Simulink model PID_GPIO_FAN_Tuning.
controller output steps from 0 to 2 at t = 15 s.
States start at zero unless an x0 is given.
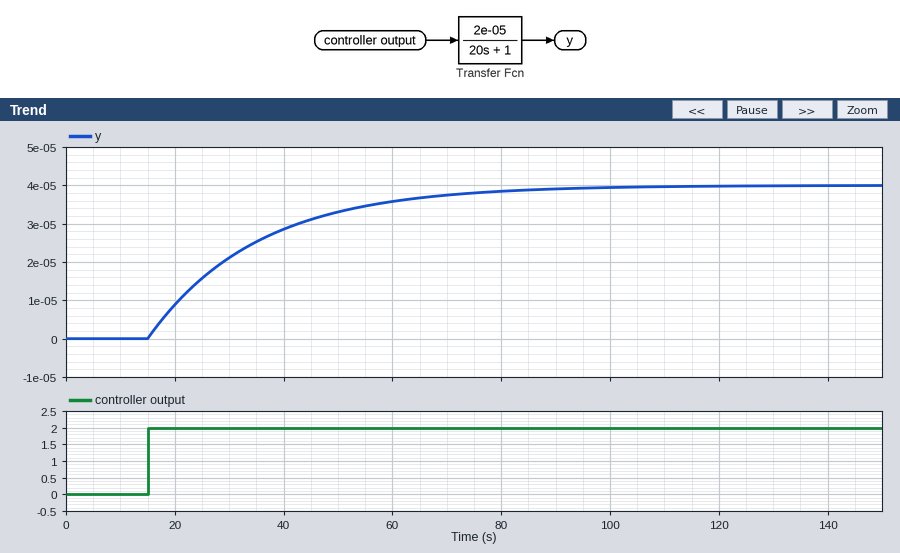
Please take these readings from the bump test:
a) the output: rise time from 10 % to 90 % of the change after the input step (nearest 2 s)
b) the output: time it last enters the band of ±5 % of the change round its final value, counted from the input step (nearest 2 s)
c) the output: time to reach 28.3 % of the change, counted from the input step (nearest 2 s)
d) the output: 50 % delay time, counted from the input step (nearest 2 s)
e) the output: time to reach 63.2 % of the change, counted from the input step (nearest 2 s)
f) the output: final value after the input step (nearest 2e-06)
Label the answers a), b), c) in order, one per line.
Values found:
a) 44 s
b) 60 s
c) 6 s
d) 14 s
e) 20 s
f) 0.000040
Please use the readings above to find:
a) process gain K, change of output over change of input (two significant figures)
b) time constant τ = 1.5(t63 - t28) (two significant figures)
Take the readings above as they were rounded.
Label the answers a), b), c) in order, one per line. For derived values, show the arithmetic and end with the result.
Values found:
a) (4e-05 - 0) / 2 = 0.000020
b) 1.5 × (20 - 6) = 21 s
